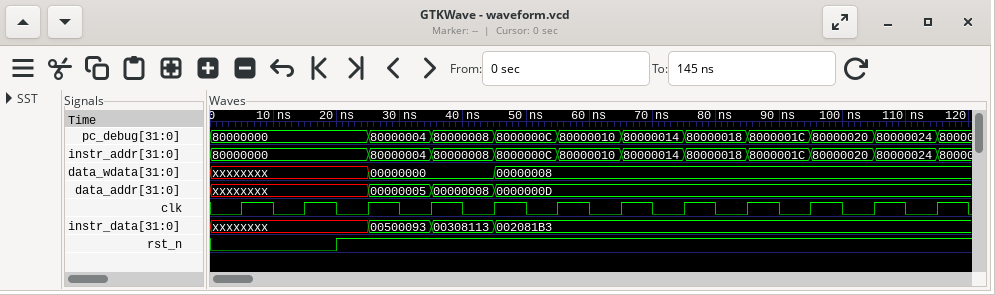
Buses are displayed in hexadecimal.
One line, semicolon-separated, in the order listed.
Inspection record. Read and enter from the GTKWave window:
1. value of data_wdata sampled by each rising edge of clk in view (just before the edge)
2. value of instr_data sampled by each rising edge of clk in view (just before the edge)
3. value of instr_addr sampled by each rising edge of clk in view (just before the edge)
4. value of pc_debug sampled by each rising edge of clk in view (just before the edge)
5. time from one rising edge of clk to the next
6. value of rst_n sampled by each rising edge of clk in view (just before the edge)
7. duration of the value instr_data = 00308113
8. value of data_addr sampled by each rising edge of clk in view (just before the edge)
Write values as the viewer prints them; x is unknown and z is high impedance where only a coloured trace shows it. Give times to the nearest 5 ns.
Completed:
xxxxxxxx, xxxxxxxx, xxxxxxxx, 00000000, 00000000, 00000008, 00000008, 00000008, 00000008, 00000008, 00000008, 00000008; xxxxxxxx, xxxxxxxx, xxxxxxxx, 00500093, 00308113, 002081B3, 002081B3, 002081B3, 002081B3, 002081B3, 002081B3, 002081B3; 80000000, 80000000, 80000000, 80000004, 80000008, 8000000C, 80000010, 80000014, 80000018, 8000001C, 80000020, 80000024; 80000000, 80000000, 80000000, 80000004, 80000008, 8000000C, 80000010, 80000014, 80000018, 8000001C, 80000020, 80000024; 10 ns; 0 0 1 1 1 1 1 1 1 1 1 1; 10 ns; xxxxxxxx, xxxxxxxx, xxxxxxxx, 00000005, 00000008, 0000000D, 0000000D, 0000000D, 0000000D, 0000000D, 0000000D, 0000000D
